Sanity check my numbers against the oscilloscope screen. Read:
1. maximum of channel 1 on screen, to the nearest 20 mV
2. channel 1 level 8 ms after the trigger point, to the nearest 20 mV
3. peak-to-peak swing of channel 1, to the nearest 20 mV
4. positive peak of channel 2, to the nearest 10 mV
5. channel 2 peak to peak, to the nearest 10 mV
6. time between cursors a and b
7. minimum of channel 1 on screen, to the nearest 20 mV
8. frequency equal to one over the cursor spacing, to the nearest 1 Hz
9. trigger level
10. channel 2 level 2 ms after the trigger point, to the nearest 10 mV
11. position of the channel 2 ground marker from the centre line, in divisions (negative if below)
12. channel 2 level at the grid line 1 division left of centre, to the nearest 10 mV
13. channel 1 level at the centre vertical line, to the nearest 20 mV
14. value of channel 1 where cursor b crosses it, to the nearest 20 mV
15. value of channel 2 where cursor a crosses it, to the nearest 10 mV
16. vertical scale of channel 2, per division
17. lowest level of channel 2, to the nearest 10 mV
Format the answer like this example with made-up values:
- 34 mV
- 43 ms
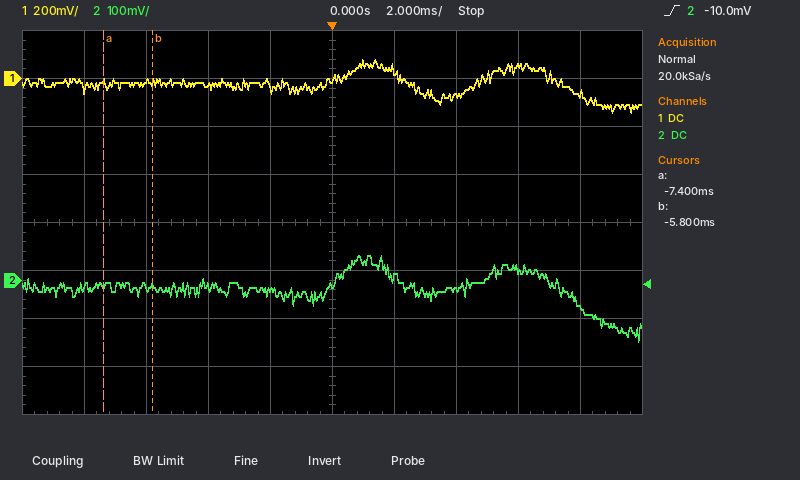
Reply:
- 80 mV
- -60 mV
- 220 mV
- 50 mV
- 180 mV
- 1.6 ms
- -140 mV
- 625 Hz
- -10.0 mV
- 0 mV
- -1.2 div
- -20 mV
- 0 mV
- -20 mV
- -10 mV
- 100 mV
- -130 mV
